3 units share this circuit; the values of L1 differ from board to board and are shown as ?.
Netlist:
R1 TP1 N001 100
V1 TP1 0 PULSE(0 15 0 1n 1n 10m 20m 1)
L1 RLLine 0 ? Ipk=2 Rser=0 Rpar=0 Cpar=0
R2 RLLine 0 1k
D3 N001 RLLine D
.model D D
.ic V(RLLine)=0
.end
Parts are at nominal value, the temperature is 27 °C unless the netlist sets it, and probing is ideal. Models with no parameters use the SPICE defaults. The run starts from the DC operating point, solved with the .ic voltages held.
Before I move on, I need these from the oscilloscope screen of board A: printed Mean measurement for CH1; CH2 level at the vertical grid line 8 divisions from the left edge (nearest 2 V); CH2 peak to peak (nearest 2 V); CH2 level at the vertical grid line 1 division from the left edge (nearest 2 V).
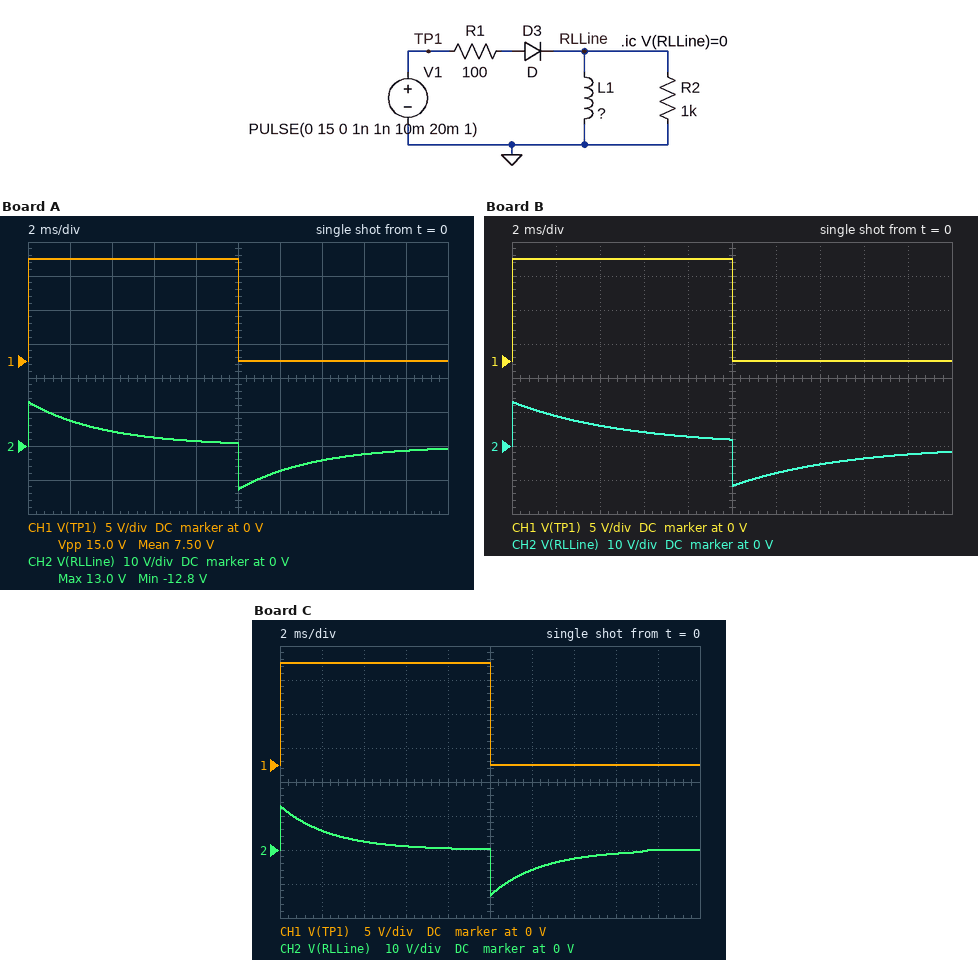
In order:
7.50 V
-2 V
26 V
8 V
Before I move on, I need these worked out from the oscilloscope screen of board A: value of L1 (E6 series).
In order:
330 mH
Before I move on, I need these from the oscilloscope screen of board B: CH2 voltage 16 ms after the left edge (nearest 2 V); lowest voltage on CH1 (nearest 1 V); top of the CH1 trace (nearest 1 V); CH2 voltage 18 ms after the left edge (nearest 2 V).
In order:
-4 V
0 V
15 V
-2 V
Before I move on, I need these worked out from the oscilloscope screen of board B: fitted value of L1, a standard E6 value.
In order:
470 mH
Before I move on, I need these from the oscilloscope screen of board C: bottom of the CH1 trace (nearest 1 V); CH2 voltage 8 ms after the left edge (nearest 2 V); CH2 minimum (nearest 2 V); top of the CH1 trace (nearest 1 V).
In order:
0 V
0 V
-14 V
15 V
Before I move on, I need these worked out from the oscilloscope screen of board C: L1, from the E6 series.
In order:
220 mH
